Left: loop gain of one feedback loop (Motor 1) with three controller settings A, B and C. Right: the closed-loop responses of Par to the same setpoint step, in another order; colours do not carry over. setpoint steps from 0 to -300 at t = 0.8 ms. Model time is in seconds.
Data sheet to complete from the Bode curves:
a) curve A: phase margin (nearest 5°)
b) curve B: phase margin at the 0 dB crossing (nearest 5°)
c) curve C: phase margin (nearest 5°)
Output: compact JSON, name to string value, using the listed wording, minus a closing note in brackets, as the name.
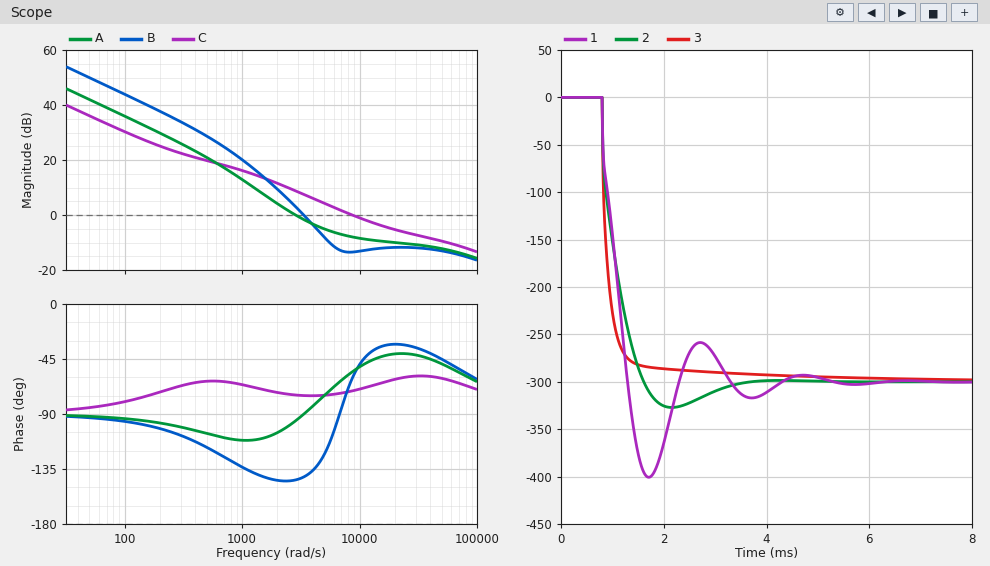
{"curve A: phase margin": "85°", "curve B: phase margin at the 0 dB crossing": "40°", "curve C: phase margin": "110°"}
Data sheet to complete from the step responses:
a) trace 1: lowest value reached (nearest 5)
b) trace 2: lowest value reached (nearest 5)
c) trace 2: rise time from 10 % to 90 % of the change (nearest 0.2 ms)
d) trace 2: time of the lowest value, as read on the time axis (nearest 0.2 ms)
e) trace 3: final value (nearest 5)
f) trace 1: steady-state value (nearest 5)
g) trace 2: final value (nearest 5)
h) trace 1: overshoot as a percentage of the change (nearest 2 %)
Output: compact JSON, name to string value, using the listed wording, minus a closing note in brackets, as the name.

{"trace 1: lowest value reached": "-400", "trace 2: lowest value reached": "-325", "trace 2: rise time from 10 % to 90 % of the change": "0.6 ms", "trace 2: time of the lowest value, as read on the time axis": "2.2 ms", "trace 3: final value": "-300", "trace 1: steady-state value": "-300", "trace 2: final value": "-300", "trace 1: overshoot as a percentage of the change": "34 %"}
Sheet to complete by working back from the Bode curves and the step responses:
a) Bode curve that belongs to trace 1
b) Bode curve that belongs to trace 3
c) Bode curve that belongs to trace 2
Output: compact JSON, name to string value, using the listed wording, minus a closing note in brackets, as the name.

{"Bode curve that belongs to trace 1": "B", "Bode curve that belongs to trace 3": "C", "Bode curve that belongs to trace 2": "A"}
